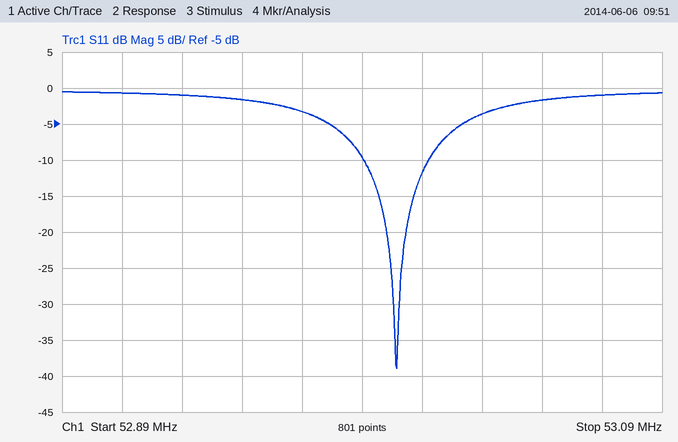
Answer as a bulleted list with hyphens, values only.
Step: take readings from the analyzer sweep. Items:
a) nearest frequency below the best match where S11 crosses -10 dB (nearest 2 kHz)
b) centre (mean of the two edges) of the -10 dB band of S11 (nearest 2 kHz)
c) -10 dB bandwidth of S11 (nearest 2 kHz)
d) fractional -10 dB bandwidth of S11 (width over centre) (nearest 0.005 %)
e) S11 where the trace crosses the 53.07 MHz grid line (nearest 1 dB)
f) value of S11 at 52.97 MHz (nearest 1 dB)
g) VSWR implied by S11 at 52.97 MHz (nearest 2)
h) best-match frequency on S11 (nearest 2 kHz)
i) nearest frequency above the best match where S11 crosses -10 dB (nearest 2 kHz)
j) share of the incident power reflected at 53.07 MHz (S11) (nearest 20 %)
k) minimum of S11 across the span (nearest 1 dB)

- 52.990 MHz
- 53.002 MHz
- 22 kHz
- 0.040 %
- -1 dB
- -3 dB
- 6
- 53.002 MHz
- 53.012 MHz
- 80 %
- -39 dB
